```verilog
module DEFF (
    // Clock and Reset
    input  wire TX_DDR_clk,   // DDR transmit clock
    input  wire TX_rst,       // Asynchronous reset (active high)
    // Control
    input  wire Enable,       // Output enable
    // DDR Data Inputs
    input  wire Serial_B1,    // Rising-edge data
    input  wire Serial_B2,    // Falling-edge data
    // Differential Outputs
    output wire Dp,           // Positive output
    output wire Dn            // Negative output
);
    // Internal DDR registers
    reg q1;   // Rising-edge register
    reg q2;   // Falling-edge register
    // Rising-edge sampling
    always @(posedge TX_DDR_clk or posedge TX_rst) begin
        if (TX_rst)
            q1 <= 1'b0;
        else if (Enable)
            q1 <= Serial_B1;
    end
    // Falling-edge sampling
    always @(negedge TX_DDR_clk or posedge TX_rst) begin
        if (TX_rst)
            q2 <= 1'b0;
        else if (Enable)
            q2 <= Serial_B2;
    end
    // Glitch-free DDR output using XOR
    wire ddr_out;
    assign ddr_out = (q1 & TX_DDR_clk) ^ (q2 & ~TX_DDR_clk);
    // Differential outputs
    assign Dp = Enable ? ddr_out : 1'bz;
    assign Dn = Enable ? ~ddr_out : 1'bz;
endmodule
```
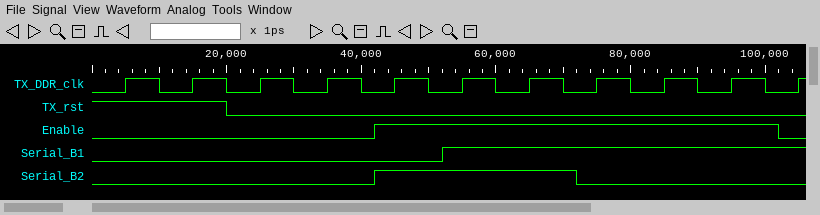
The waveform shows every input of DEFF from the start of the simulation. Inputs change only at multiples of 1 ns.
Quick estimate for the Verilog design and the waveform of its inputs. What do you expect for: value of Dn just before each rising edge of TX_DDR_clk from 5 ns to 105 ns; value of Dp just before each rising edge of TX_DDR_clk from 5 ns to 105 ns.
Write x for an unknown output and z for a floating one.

z z z z 1 0 0 0 1 1 z
z z z z 0 1 1 1 0 0 z
